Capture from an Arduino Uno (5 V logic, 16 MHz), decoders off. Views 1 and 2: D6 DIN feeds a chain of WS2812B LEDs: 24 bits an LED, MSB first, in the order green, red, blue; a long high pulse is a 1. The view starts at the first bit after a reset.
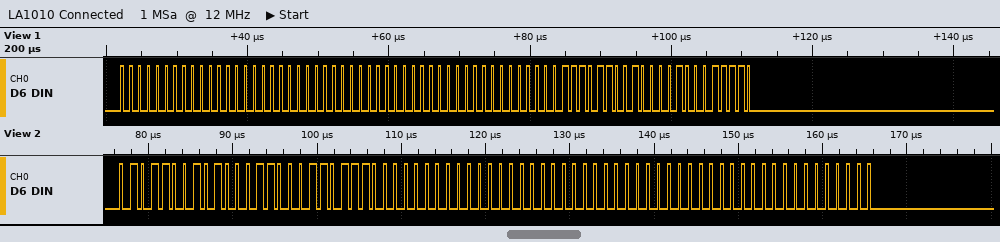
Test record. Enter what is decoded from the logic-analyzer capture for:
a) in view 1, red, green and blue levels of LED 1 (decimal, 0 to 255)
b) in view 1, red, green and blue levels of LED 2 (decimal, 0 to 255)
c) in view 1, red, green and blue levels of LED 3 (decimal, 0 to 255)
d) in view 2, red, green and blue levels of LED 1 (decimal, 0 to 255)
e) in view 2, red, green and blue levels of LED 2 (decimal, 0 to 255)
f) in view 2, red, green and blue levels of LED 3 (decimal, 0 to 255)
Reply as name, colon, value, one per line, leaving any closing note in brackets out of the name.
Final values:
in view 1, red, green and blue levels of LED 1: 0, 0, 0
in view 1, red, green and blue levels of LED 2: 0, 0, 0
in view 1, red, green and blue levels of LED 3: 33, 59, 30
in view 2, red, green and blue levels of LED 1: 70, 89, 55
in view 2, red, green and blue levels of LED 2: 0, 0, 0
in view 2, red, green and blue levels of LED 3: 0, 0, 0
